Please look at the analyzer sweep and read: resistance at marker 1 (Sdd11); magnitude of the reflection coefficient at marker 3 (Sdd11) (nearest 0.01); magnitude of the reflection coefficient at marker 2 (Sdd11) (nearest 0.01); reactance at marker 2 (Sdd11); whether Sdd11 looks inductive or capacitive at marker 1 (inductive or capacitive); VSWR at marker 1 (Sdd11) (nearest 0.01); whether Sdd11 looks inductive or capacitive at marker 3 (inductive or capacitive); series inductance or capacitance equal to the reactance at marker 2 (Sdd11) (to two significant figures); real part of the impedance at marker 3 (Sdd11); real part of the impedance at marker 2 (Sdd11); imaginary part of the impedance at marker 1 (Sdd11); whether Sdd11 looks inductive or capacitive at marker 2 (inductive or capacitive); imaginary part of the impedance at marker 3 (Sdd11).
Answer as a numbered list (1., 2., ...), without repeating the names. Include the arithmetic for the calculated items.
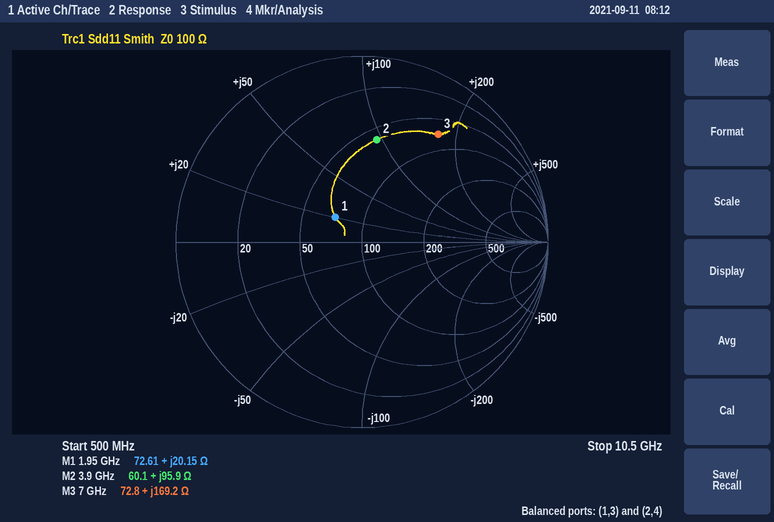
1. 72.61 Ω
2. 0.71
3. 0.56
4. +95.9 Ω
5. inductive
6. 1.49
7. inductive
8. L = 95.9 Ω/(2π × 3.9 GHz) ≈ 3.9 nH
9. 72.8 Ω
10. 60.1 Ω
11. +20.15 Ω
12. inductive
13. +169.2 Ω
